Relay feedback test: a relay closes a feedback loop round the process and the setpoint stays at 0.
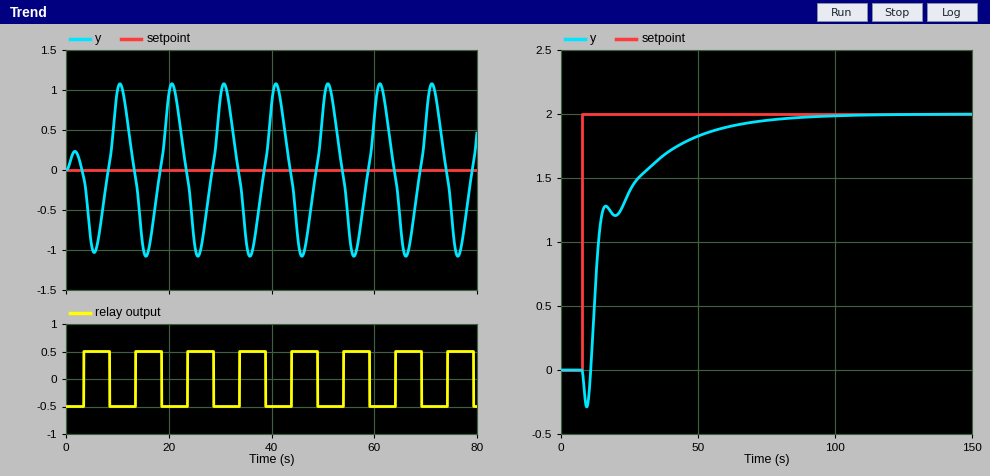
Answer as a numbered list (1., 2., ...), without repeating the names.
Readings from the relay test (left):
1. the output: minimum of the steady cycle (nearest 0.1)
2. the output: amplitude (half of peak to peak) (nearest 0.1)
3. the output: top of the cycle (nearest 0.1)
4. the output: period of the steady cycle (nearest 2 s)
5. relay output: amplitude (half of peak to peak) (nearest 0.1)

1. -1.1
2. 1.1
3. 1.1
4. 10 s
5. 0.5
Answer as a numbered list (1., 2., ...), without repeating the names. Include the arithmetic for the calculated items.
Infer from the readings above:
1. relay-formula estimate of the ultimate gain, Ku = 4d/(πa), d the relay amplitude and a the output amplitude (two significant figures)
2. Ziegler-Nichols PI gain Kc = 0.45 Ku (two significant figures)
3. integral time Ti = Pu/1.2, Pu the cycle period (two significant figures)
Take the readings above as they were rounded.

1. 4 × 0.5 / (π × 1.1) = 0.58
2. 0.45 × 0.58 = 0.26
3. 10 / 1.2 = 8.3 s
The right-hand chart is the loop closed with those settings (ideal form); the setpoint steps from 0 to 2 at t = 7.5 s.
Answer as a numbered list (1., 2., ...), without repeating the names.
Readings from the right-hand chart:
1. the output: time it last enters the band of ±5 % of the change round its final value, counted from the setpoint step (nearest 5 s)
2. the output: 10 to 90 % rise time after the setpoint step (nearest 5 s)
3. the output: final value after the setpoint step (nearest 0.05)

1. 55 s
2. 35 s
3. 2.00
